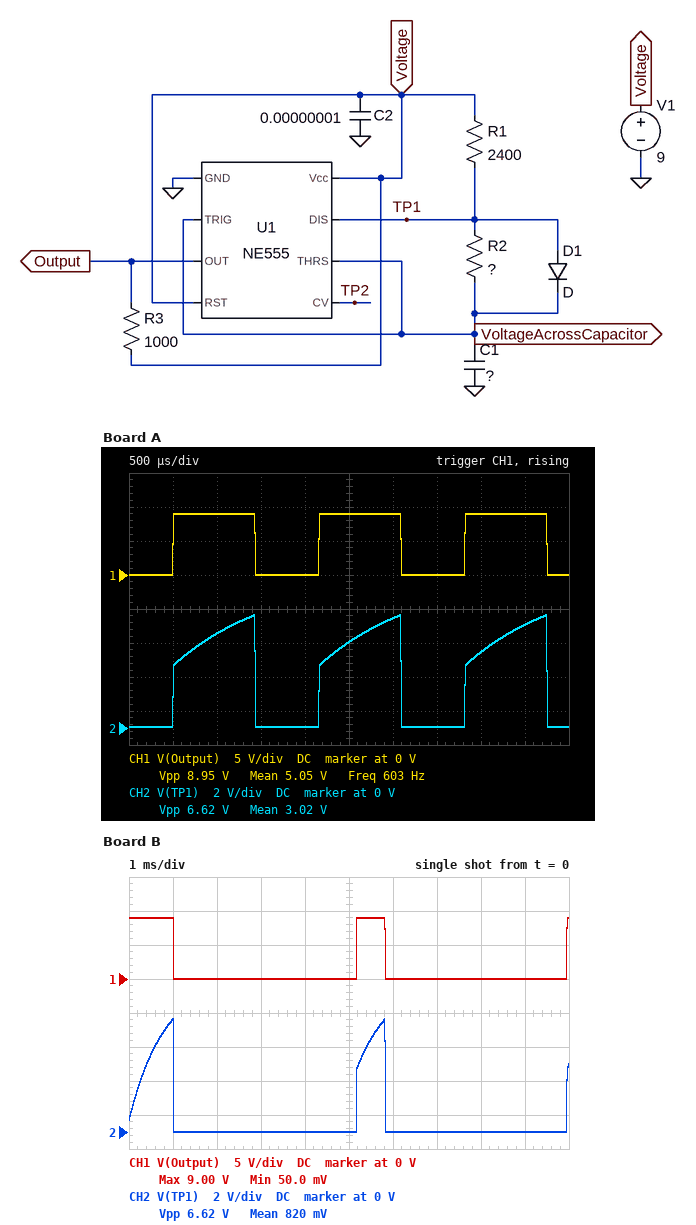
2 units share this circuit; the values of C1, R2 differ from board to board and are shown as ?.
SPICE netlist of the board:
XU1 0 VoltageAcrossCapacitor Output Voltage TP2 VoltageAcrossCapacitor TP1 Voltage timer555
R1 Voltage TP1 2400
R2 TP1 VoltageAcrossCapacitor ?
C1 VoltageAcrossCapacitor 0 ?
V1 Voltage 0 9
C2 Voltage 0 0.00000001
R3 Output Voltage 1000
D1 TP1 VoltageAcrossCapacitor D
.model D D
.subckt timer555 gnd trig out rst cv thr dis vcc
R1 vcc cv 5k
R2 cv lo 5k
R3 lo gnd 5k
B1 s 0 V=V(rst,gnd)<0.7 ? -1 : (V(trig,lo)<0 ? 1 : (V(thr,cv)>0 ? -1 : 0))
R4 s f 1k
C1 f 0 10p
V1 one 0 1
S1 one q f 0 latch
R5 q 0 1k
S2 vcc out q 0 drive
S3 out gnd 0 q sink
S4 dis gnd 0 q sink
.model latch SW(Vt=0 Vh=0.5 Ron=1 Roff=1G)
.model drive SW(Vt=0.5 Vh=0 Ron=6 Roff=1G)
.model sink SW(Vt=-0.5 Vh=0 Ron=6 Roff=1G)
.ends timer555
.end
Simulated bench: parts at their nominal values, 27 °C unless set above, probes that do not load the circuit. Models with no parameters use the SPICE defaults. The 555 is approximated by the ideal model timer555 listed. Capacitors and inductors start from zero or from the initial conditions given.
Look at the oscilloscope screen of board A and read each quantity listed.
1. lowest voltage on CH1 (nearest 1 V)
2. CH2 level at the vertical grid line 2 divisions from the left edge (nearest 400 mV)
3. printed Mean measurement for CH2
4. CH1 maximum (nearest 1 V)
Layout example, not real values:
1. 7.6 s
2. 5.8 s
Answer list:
1. 0 V
2. 5.6 V
3. 3.02 V
4. 9 V
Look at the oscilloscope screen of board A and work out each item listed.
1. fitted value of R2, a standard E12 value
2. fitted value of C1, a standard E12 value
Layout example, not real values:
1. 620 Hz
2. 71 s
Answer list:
1. 2.2 kΩ
2. 470 nF
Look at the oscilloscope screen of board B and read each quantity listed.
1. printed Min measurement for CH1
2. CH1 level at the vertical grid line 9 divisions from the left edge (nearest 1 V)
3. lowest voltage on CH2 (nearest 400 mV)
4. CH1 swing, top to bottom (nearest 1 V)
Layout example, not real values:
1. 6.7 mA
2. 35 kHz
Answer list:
1. 50.0 mV
2. 0 V
3. 0 V
4. 9 V
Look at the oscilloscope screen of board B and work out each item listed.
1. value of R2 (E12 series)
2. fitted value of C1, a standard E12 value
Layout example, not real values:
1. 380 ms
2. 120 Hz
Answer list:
1. 18 kΩ
2. 330 nF
